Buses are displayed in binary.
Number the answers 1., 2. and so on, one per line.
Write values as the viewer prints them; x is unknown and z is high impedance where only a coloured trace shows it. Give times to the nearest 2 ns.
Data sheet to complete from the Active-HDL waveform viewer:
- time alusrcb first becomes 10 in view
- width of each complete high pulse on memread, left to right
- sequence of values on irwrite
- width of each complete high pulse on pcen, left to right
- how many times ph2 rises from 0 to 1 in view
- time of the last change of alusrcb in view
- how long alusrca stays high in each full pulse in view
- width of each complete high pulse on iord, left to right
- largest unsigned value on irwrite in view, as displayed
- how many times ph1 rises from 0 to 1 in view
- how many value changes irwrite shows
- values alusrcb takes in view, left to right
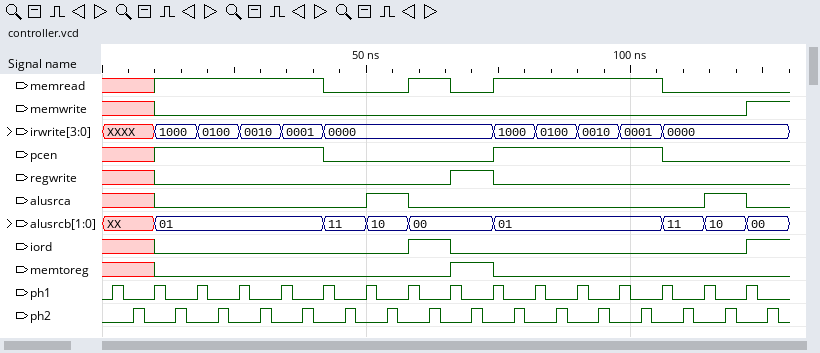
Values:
1. 50 ns
2. 8 ns, 32 ns
3. XXXX, 1000, 0100, 0010, 0001, 0000, 1000, 0100, 0010, 0001, 0000
4. 32 ns
5. 16
6. 122 ns
7. 8 ns, 8 ns
8. 8 ns
9. 1000
10. 16
11. 10
12. XX, 01, 11, 10, 00, 01, 11, 10, 00
